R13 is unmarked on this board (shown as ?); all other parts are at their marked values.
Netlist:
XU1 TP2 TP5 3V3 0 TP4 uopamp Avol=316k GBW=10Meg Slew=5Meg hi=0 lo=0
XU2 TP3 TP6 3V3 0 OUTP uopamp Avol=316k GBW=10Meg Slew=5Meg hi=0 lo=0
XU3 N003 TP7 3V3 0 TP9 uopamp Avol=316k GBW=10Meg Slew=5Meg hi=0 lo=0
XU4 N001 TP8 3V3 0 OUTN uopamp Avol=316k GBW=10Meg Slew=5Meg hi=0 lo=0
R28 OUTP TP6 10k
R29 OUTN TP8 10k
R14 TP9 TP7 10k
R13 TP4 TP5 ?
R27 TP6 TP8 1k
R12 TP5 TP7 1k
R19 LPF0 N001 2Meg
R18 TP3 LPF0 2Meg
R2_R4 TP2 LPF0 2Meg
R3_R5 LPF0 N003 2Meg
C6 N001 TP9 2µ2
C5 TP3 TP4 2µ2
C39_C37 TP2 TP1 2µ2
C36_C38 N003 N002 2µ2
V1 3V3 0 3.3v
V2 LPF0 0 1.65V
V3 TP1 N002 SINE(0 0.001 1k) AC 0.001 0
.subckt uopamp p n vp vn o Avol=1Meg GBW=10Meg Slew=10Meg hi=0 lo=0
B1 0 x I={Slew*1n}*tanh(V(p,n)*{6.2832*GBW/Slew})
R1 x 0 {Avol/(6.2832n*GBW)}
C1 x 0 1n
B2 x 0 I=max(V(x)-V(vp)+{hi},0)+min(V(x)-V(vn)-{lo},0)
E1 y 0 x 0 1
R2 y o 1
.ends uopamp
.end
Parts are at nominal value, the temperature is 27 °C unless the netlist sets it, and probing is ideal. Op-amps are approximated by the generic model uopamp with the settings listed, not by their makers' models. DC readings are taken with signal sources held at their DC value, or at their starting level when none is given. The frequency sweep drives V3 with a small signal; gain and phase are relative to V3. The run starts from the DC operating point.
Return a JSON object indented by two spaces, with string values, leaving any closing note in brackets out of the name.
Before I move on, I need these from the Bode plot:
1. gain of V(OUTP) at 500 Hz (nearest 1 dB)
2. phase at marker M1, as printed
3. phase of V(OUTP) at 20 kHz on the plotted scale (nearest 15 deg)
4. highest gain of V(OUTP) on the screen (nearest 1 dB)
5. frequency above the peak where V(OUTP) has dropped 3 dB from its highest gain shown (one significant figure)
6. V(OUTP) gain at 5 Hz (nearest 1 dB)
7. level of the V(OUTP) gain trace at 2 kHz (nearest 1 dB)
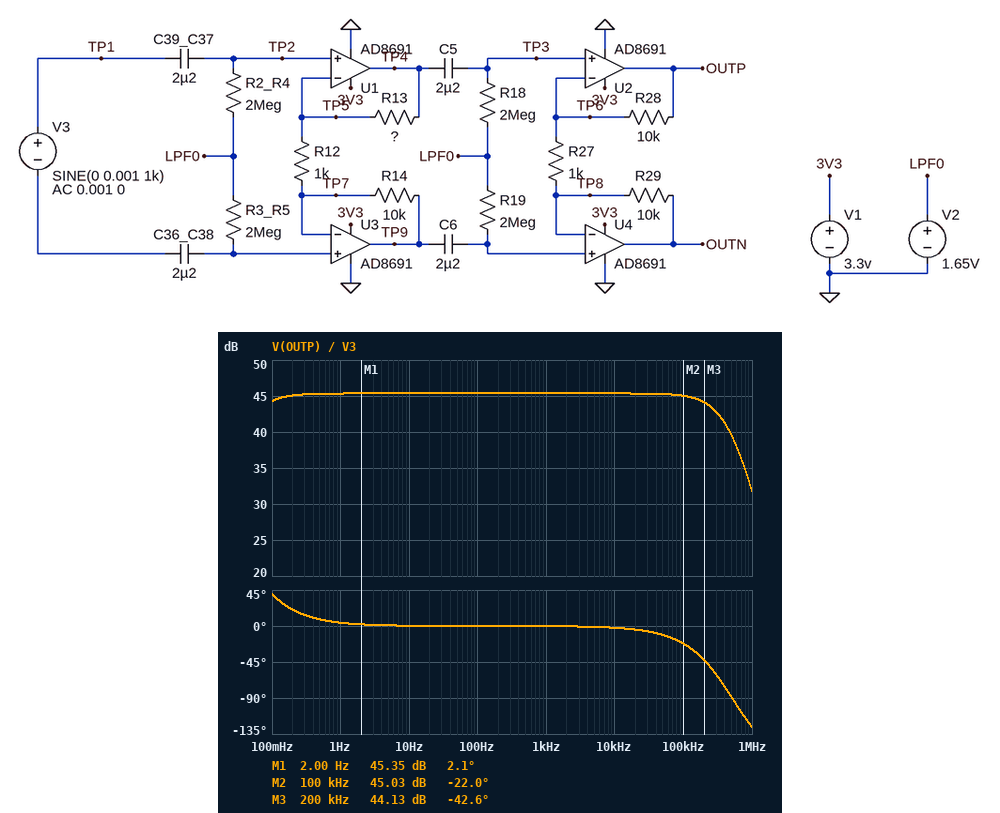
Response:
{
  "gain of V(OUTP) at 500 Hz": "45 dB",
  "phase at marker M1, as printed": "2.1 deg",
  "phase of V(OUTP) at 20 kHz on the plotted scale": "0 deg",
  "highest gain of V(OUTP) on the screen": "45 dB",
  "frequency above the peak where V(OUTP) has dropped 3 dB from its highest gain shown": "300 kHz",
  "V(OUTP) gain at 5 Hz": "45 dB",
  "level of the V(OUTP) gain trace at 2 kHz": "45 dB"
}
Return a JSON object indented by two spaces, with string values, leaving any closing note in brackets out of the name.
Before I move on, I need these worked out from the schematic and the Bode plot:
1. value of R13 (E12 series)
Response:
{
  "value of R13": "6.8 kΩ"
}
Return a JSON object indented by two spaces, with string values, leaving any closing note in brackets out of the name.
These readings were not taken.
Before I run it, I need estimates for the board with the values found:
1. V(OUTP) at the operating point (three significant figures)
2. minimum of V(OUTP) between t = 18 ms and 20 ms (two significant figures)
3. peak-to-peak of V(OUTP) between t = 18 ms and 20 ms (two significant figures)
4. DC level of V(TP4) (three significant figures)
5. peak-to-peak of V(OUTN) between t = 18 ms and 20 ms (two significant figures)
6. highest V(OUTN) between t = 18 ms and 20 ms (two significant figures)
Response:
{
  "V(OUTP) at the operating point": "1.65 V",
  "minimum of V(OUTP) between t = 18 ms and 20 ms": "1.5 V",
  "peak-to-peak of V(OUTP) between t = 18 ms and 20 ms": "370 mV",
  "DC level of V(TP4)": "1.65 V",
  "peak-to-peak of V(OUTN) between t = 18 ms and 20 ms": "380 mV",
  "highest V(OUTN) between t = 18 ms and 20 ms": "1.8 V"
}
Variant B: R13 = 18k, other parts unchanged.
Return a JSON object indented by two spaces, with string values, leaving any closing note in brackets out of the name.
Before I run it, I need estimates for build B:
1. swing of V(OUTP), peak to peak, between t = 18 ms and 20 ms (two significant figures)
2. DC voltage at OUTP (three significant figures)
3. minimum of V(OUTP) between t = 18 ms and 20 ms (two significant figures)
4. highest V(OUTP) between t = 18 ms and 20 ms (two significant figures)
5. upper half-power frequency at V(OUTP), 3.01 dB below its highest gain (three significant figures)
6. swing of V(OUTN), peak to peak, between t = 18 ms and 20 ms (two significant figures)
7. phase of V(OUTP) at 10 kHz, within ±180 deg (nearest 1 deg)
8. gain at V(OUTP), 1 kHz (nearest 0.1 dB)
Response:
{
  "swing of V(OUTP), peak to peak, between t = 18 ms and 20 ms": "620 mV",
  "DC voltage at OUTP": "1.65 V",
  "minimum of V(OUTP) between t = 18 ms and 20 ms": "1.3 V",
  "highest V(OUTP) between t = 18 ms and 20 ms": "2.0 V",
  "upper half-power frequency at V(OUTP), 3.01 dB below its highest gain": "256 kHz",
  "swing of V(OUTN), peak to peak, between t = 18 ms and 20 ms": "600 mV",
  "phase of V(OUTP) at 10 kHz, within ±180 deg": "-3 deg",
  "gain at V(OUTP), 1 kHz": "49.8 dB"
}
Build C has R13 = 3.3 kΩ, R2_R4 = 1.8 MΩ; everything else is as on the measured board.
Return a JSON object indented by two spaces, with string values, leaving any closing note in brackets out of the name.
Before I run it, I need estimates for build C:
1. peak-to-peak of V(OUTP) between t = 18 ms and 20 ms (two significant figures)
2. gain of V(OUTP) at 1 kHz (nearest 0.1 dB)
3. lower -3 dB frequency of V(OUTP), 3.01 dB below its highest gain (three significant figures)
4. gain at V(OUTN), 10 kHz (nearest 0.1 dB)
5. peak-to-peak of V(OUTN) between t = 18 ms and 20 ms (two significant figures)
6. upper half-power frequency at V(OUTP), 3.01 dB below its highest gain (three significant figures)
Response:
{
  "peak-to-peak of V(OUTP) between t = 18 ms and 20 ms": "290 mV",
  "gain of V(OUTP) at 1 kHz": "43.3 dB",
  "lower -3 dB frequency of V(OUTP), 3.01 dB below its highest gain": "57.7 mHz",
  "gain at V(OUTN), 10 kHz": "43.7 dB",
  "peak-to-peak of V(OUTN) between t = 18 ms and 20 ms": "310 mV",
  "upper half-power frequency at V(OUTP), 3.01 dB below its highest gain": "361 kHz"
}
